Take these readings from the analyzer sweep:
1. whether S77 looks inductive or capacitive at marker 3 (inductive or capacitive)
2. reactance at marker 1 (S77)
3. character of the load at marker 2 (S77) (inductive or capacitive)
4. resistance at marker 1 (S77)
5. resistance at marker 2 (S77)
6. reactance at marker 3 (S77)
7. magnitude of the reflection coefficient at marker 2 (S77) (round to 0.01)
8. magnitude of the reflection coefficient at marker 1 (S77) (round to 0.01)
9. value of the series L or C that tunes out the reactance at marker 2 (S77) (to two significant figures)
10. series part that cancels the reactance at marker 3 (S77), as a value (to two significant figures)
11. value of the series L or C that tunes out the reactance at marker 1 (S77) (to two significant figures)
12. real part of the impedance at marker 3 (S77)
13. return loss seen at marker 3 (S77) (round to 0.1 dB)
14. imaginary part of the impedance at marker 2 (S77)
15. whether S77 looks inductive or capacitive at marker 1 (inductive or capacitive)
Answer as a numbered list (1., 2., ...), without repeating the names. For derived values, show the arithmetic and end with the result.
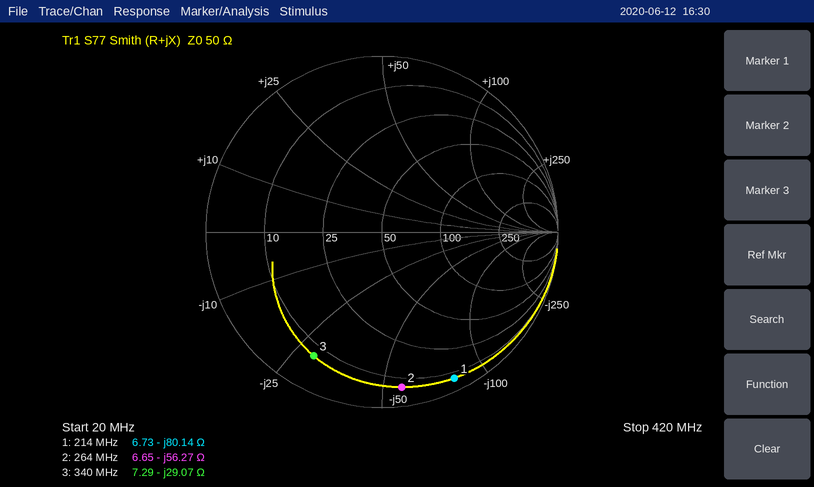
1. capacitive
2. -80.14 Ω
3. capacitive
4. 6.73 Ω
5. 6.65 Ω
6. -29.07 Ω
7. 0.89
8. 0.93
9. L = 56.27 Ω/(2π × 264 MHz) ≈ 34 nH
10. L = 29.07 Ω/(2π × 340 MHz) ≈ 14 nH
11. L = 80.14 Ω/(2π × 214 MHz) ≈ 60 nH
12. 7.29 Ω
13. 1.9 dB
14. -56.27 Ω
15. capacitive
